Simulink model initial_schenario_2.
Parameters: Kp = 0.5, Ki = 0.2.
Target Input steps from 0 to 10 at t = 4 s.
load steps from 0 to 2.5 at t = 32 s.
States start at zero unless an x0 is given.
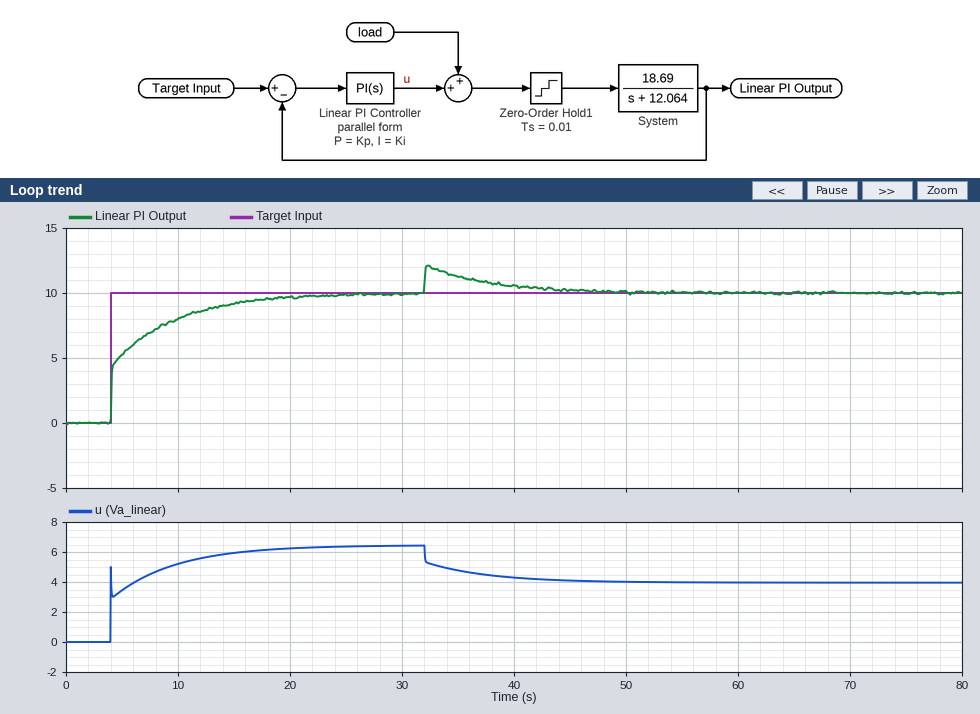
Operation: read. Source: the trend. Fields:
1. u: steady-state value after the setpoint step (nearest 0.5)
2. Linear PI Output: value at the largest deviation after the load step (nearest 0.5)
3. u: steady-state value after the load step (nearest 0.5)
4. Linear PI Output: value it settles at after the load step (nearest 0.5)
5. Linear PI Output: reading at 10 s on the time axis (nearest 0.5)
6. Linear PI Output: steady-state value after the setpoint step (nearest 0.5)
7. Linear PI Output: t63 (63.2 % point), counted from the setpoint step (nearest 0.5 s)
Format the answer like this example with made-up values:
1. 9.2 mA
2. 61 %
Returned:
1. 6.5
2. 12.0
3. 4.0
4. 10.0
5. 8.0
6. 10.0
7. 2.5 s
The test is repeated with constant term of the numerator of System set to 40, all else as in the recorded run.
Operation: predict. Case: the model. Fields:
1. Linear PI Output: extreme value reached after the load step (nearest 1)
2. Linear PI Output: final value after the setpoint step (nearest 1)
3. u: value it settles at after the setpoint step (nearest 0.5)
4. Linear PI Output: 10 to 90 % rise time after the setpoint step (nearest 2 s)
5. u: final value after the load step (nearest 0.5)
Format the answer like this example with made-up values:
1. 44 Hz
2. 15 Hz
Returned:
1. 13
2. 10
3. 3.0
4. 6 s
5. 0.5
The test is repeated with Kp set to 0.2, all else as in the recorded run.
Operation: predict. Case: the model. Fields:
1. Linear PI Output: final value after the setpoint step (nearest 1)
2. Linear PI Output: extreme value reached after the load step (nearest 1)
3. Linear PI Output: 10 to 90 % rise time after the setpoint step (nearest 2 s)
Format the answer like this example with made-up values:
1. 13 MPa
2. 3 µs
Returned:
1. 10
2. 13
3. 8 s
